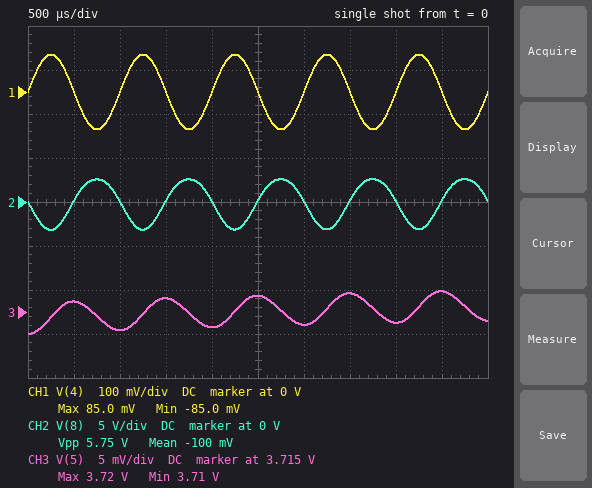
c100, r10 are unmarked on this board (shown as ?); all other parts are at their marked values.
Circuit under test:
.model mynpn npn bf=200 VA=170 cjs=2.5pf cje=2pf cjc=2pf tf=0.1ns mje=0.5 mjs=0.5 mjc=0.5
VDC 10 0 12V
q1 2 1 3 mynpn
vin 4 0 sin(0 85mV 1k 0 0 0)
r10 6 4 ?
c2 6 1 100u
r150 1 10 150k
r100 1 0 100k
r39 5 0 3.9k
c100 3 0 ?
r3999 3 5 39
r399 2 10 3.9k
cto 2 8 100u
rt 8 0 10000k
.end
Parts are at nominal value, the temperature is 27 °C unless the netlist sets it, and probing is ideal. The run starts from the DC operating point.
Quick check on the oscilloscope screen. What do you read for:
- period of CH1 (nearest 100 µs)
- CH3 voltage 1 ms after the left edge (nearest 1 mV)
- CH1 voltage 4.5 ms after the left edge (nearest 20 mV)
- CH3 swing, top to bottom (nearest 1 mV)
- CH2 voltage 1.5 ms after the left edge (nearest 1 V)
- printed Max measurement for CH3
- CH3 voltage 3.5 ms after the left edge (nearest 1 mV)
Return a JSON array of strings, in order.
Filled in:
["1.0 ms", "3.713 V", "0 V", "5 mV", "0 V", "3.72 V", "3.717 V"]
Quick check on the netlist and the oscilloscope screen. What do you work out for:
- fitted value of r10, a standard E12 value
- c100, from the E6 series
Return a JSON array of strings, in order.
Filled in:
["15 kΩ", "68 µF"]
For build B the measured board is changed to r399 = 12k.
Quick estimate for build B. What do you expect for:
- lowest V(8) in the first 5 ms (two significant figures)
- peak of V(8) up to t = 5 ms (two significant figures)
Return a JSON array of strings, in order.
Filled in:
["-8.5 mV", "13 mV"]
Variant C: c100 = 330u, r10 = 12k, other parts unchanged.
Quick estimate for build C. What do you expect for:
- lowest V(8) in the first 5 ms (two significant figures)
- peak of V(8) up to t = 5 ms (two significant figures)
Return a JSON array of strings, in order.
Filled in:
["-3.9 V", "2.8 V"]
